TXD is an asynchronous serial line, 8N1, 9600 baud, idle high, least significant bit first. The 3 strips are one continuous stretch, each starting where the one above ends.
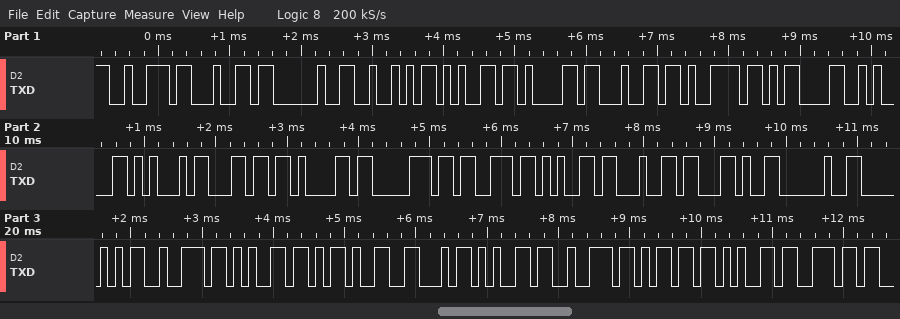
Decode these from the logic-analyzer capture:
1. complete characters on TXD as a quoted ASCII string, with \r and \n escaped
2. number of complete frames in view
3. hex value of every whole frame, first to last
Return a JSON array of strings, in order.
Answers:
["\"rd Ready\\r\\nElapsed, Pre-Fermen\"", "29", "72 64 20 52 65 61 64 79 0D 0A 45 6C 61 70 73 65 64 2C 20 50 72 65 2D 46 65 72 6D 65 6E"]
